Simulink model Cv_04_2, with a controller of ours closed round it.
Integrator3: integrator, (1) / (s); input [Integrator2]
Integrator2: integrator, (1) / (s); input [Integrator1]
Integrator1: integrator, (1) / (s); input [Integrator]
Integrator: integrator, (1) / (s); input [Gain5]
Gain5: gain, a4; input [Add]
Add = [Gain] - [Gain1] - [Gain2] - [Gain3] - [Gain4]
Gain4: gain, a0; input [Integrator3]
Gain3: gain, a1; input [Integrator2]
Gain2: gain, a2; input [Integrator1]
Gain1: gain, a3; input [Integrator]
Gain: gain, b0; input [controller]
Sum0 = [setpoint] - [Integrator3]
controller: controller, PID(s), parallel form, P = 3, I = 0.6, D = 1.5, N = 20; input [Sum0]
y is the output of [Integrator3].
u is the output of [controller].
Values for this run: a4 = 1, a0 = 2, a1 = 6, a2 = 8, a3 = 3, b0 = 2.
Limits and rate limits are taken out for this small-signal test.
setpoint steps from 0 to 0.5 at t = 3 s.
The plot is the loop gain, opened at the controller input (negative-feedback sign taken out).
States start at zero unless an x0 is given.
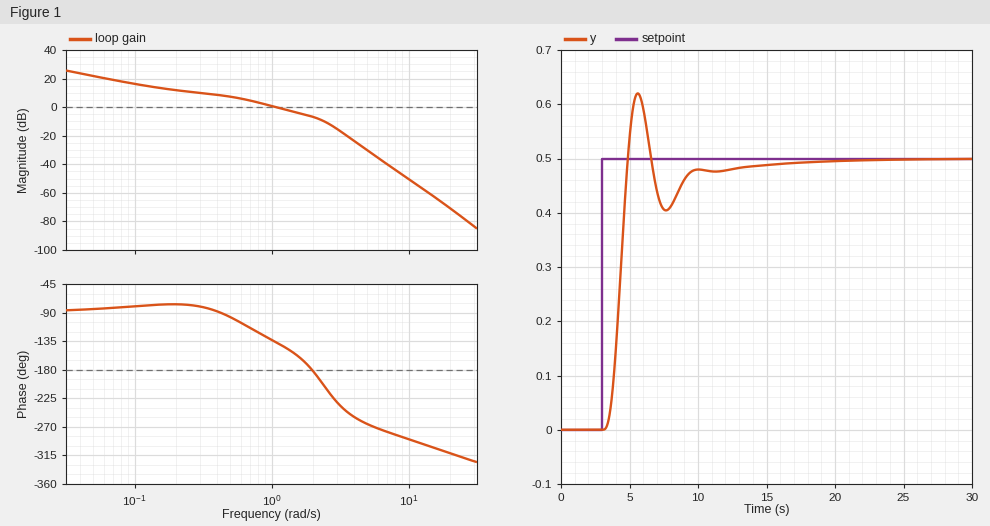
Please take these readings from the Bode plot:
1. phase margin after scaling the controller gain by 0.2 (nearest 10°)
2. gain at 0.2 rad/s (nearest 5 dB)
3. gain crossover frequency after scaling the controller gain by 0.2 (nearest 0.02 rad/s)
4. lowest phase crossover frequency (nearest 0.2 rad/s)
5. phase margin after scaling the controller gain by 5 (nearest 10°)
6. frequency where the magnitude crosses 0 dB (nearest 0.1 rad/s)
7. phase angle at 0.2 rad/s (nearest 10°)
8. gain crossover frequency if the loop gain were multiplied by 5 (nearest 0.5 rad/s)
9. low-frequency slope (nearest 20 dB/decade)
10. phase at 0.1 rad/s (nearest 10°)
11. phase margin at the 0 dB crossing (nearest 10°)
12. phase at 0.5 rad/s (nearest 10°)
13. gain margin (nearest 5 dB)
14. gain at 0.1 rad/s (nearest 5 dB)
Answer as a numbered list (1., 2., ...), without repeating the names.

1. 100°
2. 10 dB
3. 0.14 rad/s
4. 2.0 rad/s
5. -50°
6. 1.1 rad/s
7. -80°
8. 3.0 rad/s
9. -20 dB/decade
10. -80°
11. 40°
12. -100°
13. 5 dB
14. 15 dB
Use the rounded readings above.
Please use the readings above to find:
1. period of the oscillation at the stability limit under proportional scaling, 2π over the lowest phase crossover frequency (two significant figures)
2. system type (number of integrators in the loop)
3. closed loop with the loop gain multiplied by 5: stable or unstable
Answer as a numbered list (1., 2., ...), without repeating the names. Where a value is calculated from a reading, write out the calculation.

1. 2π / 2 = 3.1 s
2. 1
3. unstable
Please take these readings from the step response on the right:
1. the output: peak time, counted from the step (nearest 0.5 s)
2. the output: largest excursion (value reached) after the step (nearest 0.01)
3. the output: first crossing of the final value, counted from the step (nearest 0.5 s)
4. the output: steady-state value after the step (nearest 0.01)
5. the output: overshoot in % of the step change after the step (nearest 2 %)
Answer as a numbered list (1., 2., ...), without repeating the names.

1. 2.5 s
2. 0.62
3. 2.0 s
4. 0.50
5. 24 %
